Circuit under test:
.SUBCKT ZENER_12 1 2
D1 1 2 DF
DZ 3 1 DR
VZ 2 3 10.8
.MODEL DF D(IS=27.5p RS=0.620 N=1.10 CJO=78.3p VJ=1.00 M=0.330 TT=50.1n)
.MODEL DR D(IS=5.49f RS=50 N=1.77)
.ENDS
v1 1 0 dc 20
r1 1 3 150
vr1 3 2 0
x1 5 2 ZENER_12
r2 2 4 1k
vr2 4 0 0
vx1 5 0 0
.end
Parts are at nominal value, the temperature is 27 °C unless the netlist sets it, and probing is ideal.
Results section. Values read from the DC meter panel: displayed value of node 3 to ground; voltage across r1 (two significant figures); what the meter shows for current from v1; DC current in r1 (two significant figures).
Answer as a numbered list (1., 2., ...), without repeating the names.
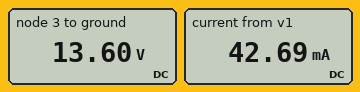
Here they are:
1. 13.60 V
2. 6.4 V
3. 42.69 mA
4. 43 mA
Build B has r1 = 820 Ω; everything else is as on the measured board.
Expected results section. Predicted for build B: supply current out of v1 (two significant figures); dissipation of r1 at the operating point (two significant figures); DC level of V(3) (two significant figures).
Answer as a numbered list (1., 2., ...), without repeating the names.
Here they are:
1. 11 mA
2. 99 mW
3. 11 V
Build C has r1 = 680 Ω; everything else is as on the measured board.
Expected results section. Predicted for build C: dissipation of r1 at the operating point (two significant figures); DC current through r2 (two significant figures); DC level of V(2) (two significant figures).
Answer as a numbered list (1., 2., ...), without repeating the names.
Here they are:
1. 97 mW
2. 12 mA
3. 12 V
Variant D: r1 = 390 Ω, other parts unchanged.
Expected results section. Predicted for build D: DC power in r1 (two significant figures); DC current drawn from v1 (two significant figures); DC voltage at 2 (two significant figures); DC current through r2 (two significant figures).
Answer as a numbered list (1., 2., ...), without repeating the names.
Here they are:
1. 150 mW
2. 19 mA
3. 12 V
4. 12 mA
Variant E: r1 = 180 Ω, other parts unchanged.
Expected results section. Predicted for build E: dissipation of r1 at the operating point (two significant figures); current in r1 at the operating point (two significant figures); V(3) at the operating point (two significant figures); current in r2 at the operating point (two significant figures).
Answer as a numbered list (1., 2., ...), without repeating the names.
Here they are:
1. 250 mW
2. 37 mA
3. 13 V
4. 13 mA
